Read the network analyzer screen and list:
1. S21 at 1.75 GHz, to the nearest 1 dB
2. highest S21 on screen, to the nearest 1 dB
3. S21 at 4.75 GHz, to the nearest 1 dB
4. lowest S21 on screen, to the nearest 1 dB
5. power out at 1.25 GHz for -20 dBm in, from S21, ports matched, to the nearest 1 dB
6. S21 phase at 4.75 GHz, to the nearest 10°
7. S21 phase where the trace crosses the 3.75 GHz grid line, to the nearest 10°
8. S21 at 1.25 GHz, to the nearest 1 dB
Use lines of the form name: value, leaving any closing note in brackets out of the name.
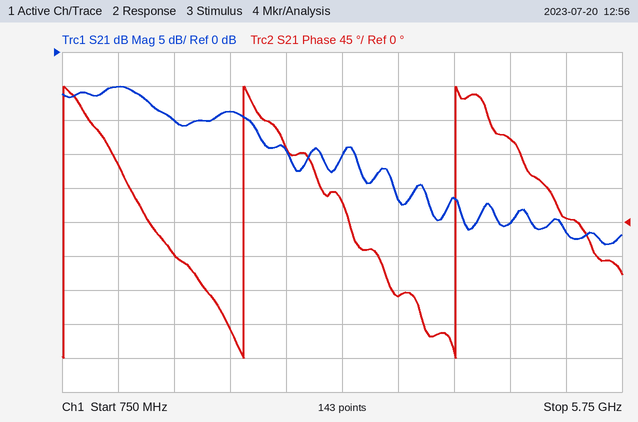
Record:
S21 at 1.75 GHz, to the nearest 1 dB: -10 dB
highest S21 on screen, to the nearest 1 dB: -5 dB
S21 at 4.75 GHz, to the nearest 1 dB: -25 dB
lowest S21 on screen, to the nearest 1 dB: -28 dB
power out at 1.25 GHz for -20 dBm in, from S21, ports matched, to the nearest 1 dB: -25 dBm
S21 phase at 4.75 GHz, to the nearest 10°: 110°
S21 phase where the trace crosses the 3.75 GHz grid line, to the nearest 10°: -100°
S21 at 1.25 GHz, to the nearest 1 dB: -5 dB
